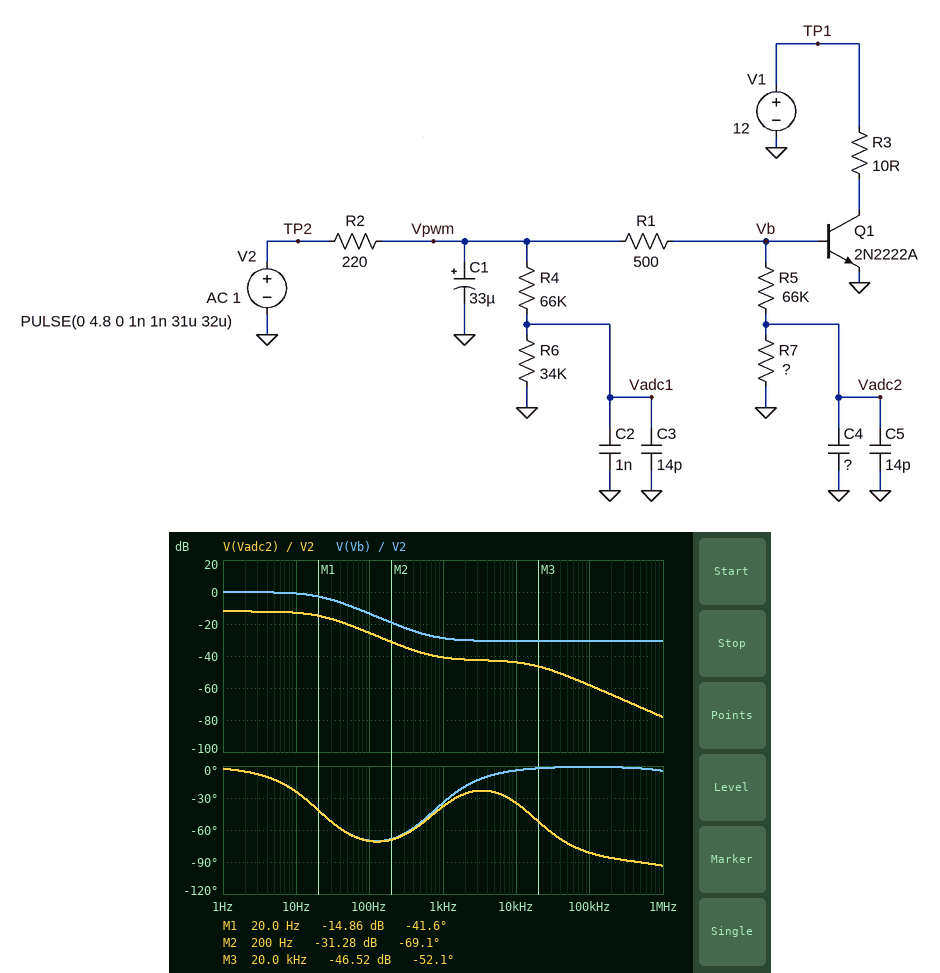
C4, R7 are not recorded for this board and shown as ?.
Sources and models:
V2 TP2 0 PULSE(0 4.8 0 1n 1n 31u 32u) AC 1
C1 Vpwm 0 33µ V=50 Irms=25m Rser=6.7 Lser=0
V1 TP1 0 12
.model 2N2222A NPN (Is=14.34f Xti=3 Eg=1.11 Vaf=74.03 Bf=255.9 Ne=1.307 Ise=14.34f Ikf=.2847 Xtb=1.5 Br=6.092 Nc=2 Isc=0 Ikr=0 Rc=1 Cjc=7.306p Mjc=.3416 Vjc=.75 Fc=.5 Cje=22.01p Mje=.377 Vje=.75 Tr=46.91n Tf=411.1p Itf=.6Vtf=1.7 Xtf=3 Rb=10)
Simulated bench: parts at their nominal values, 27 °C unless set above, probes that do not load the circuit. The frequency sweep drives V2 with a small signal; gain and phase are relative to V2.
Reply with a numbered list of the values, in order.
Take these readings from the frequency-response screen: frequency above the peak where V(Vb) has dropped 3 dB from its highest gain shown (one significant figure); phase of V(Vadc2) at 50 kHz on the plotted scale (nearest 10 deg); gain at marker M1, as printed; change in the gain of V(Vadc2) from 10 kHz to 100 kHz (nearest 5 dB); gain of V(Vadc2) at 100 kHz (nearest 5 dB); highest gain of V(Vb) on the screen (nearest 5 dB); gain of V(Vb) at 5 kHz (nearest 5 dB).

1. 20 Hz
2. -70 deg
3. -14.86 dB
4. -15 dB
5. -60 dB
6. 0 dB
7. -30 dB
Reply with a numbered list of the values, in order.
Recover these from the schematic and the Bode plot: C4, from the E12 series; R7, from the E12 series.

1. 560 pF
2. 22 kΩ
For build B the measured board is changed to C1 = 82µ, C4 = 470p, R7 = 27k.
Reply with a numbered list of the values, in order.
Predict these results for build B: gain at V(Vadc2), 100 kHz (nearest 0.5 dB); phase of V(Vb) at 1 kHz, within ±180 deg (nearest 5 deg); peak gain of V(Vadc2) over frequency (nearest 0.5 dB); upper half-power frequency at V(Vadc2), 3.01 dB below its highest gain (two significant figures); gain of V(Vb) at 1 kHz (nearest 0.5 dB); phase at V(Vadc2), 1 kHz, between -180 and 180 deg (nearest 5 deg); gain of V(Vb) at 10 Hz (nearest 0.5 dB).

1. -57.0 dB
2. -15 deg
3. -11.0 dB
4. 8.6 Hz
5. -30.5 dB
6. -20 deg
7. -4.0 dB
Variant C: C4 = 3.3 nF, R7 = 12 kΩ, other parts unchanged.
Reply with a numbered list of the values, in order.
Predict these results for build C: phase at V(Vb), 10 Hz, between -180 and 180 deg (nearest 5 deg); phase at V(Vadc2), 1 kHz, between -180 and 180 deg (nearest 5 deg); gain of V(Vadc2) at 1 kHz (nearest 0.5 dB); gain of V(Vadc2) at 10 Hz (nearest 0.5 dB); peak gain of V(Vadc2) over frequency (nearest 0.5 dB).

1. -25 deg
2. -45 deg
3. -45.5 dB
4. -17.0 dB
5. -16.5 dB
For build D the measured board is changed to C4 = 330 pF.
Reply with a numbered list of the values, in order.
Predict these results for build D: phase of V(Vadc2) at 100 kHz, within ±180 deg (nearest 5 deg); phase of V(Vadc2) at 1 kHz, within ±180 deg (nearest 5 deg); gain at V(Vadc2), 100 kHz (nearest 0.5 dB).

1. -75 deg
2. -35 deg
3. -54.0 dB
